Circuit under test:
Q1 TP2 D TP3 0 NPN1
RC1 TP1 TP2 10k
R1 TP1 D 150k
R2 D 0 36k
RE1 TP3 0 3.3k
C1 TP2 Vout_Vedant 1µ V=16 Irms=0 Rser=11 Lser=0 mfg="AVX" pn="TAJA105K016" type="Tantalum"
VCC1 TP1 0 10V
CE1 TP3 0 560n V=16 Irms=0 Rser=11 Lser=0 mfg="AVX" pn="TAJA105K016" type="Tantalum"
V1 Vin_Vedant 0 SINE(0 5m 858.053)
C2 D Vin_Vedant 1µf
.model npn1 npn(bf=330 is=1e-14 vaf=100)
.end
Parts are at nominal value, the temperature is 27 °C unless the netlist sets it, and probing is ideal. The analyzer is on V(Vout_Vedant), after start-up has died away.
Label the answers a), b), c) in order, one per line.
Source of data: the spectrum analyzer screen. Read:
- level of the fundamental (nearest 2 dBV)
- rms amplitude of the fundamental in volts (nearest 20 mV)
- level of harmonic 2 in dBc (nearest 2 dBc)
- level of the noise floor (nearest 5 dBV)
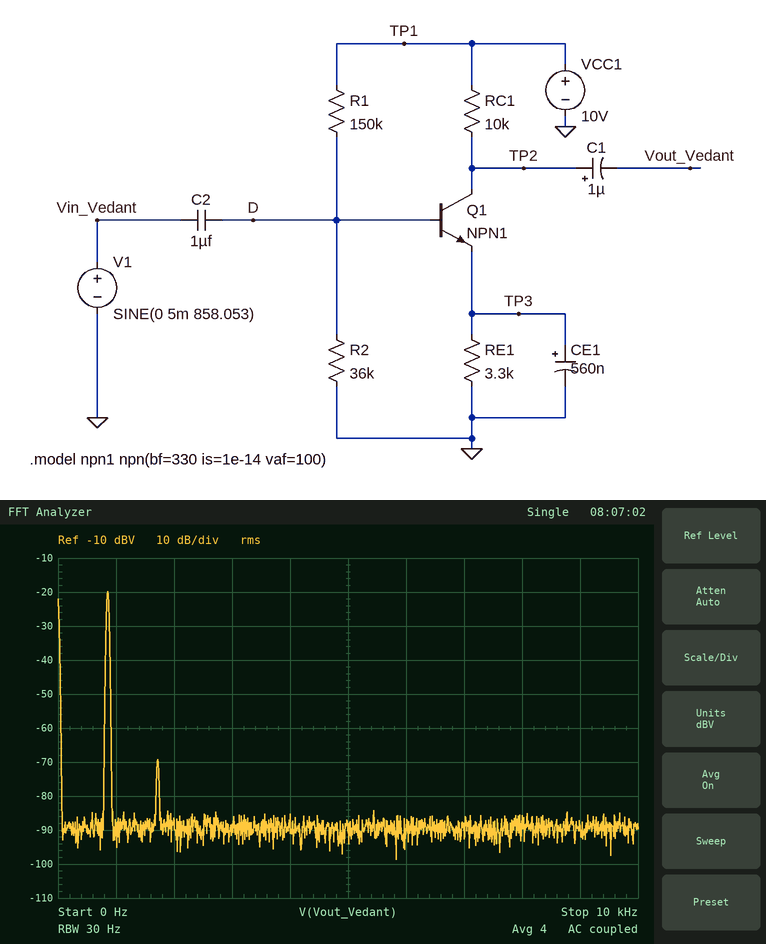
a) -20 dBV
b) 100 mV
c) -50 dBc
d) -90 dBV
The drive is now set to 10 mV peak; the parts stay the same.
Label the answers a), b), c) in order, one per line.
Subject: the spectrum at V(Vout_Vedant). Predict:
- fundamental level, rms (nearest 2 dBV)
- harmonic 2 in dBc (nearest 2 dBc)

a) -14 dBV
b) -44 dBc
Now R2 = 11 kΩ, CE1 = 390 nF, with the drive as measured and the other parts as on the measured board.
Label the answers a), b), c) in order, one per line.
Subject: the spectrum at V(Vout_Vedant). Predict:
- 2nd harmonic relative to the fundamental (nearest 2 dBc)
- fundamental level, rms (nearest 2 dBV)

a) -30 dBc
b) -28 dBV
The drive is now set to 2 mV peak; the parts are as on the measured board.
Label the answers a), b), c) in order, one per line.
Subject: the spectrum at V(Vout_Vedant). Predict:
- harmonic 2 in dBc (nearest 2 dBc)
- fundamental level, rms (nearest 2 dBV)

a) -58 dBc
b) -28 dBV
